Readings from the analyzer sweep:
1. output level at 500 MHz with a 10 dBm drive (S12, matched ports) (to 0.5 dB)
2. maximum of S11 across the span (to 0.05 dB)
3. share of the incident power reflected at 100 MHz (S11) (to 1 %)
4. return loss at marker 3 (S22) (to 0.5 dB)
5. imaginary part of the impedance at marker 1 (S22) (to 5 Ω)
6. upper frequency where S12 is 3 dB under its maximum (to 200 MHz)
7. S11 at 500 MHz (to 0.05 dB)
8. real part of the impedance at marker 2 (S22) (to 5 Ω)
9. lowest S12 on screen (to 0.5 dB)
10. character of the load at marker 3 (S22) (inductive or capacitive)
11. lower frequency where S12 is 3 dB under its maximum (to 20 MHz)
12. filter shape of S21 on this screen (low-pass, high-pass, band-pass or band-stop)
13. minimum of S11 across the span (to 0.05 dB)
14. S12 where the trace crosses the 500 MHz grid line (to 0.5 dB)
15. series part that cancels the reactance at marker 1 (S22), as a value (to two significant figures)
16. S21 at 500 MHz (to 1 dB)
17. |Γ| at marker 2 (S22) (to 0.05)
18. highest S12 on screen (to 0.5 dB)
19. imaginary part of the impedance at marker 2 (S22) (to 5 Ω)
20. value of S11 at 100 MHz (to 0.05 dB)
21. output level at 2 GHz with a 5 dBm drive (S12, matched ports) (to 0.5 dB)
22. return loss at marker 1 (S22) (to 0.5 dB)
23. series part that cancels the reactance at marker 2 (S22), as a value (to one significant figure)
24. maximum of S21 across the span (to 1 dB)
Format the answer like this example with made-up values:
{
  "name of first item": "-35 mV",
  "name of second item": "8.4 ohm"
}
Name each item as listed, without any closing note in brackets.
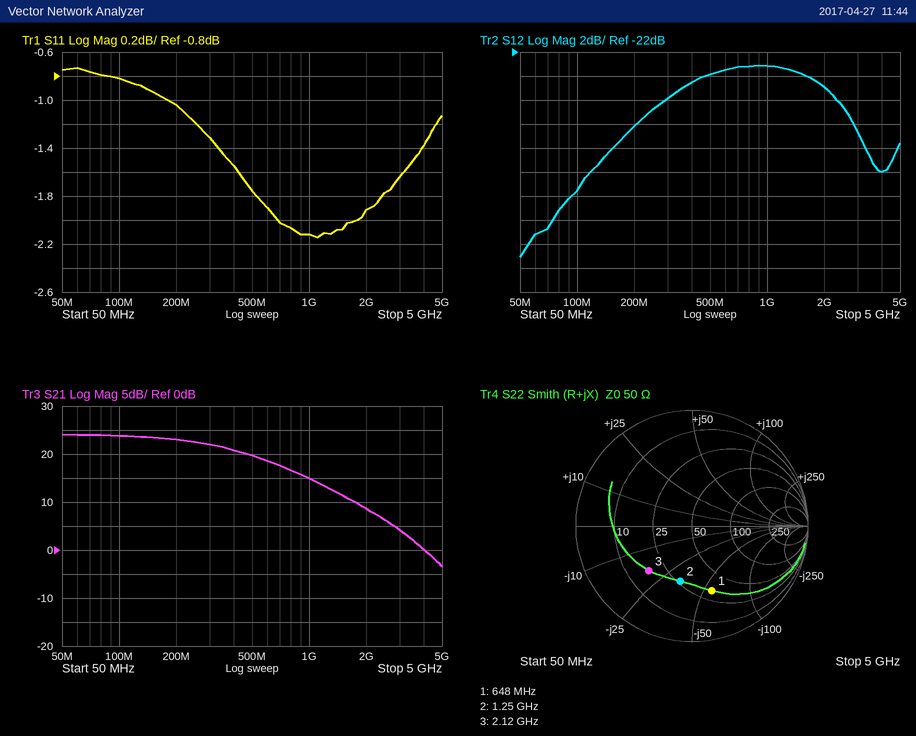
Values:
{
  "output level at 500 MHz with a 10 dBm drive (S12, matched ports)": "-14.0 dBm",
  "maximum of S11 across the span": "-0.75 dB",
  "share of the incident power reflected at 100 MHz (S11)": "83 %",
  "return loss at marker 3 (S22)": "5.5 dB",
  "imaginary part of the impedance at marker 1 (S22)": "-55 Ω",
  "upper frequency where S12 is 3 dB under its maximum": "2.4 GHz",
  "S11 at 500 MHz": "-1.75 dB",
  "real part of the impedance at marker 2 (S22)": "25 Ω",
  "lowest S12 on screen": "-39.0 dB",
  "character of the load at marker 3 (S22)": "capacitive",
  "lower frequency where S12 is 3 dB under its maximum": "280 MHz",
  "filter shape of S21 on this screen": "low-pass",
  "minimum of S11 across the span": "-2.15 dB",
  "S12 where the trace crosses the 500 MHz grid line": "-24.0 dB",
  "series part that cancels the reactance at marker 1 (S22), as a value": "14 nH",
  "S21 at 500 MHz": "20 dB",
  "|Γ| at marker 2 (S22)": "0.50",
  "highest S12 on screen": "-23.0 dB",
  "imaginary part of the impedance at marker 2 (S22)": "-35 Ω",
  "value of S11 at 100 MHz": "-0.80 dB",
  "output level at 2 GHz with a 5 dBm drive (S12, matched ports)": "-20.0 dBm",
  "return loss at marker 1 (S22)": "4.5 dB",
  "series part that cancels the reactance at marker 2 (S22), as a value": "4 nH",
  "maximum of S21 across the span": "24 dB"
}
